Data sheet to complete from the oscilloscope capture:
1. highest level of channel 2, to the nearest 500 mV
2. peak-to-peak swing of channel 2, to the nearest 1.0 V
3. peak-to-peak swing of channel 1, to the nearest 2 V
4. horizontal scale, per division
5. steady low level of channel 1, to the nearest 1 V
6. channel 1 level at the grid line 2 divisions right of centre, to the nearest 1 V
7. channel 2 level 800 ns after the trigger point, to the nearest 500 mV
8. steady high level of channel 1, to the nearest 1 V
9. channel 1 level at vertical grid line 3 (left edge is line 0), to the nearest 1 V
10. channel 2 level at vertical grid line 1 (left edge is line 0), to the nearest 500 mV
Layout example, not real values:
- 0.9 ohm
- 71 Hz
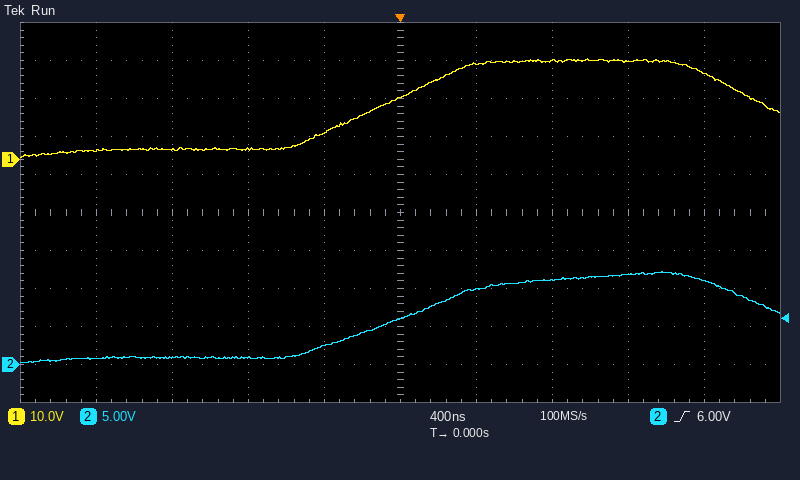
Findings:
- 12.0 V
- 12.0 V
- 26 V
- 400 ns
- 3 V
- 26 V
- 11.0 V
- 26 V
- 3 V
- 1.0 V
